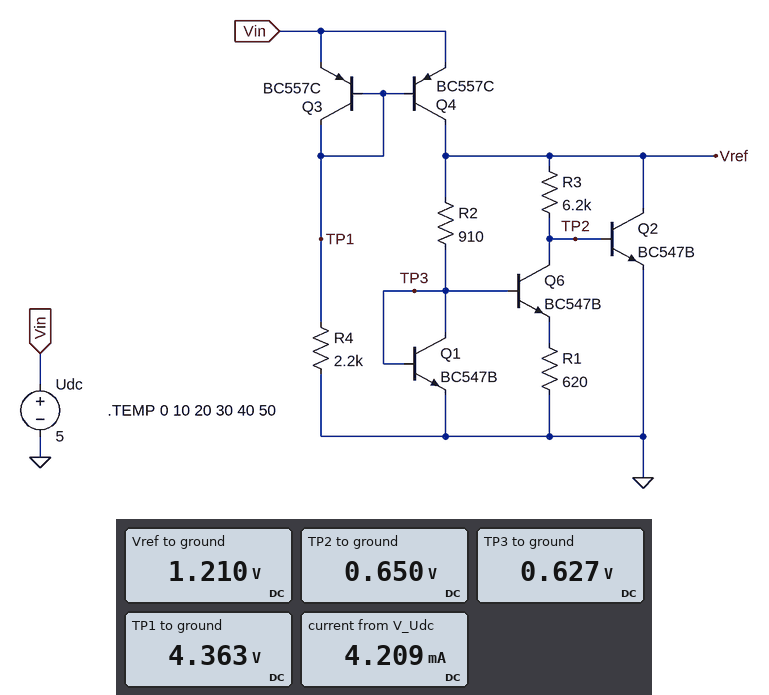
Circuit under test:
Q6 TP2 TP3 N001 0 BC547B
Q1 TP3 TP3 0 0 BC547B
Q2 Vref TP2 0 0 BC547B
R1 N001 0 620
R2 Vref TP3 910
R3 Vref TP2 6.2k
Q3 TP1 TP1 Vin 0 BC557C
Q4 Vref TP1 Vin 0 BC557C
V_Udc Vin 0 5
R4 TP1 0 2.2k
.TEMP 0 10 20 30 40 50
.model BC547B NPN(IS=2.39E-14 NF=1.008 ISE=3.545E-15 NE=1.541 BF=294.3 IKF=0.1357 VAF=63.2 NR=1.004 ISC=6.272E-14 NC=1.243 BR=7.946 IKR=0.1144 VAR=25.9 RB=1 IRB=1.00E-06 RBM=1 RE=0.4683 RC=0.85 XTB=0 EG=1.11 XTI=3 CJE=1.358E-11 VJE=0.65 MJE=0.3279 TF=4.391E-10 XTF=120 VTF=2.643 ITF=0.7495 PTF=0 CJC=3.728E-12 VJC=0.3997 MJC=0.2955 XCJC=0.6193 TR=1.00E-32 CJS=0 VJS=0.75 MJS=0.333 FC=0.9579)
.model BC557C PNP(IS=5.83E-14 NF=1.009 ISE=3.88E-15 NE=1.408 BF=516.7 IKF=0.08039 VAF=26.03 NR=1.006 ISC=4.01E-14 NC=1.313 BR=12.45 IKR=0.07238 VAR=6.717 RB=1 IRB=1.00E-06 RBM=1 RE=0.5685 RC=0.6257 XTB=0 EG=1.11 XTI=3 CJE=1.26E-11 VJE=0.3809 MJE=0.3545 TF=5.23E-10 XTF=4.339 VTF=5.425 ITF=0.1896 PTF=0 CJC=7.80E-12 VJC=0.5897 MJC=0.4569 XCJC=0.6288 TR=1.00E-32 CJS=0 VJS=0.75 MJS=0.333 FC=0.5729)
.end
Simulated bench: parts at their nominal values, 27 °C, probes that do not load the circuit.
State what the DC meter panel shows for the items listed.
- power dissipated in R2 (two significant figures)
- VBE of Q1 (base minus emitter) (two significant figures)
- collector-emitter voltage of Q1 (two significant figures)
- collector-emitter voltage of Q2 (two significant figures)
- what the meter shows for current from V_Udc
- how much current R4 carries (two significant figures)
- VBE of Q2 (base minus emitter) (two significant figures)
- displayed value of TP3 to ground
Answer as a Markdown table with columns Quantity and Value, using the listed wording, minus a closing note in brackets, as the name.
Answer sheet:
| Quantity | Value |
|---|---|
| power dissipated in R2 | 370 µW |
| VBE of Q1 (base minus emitter) | 630 mV |
| collector-emitter voltage of Q1 | 630 mV |
| collector-emitter voltage of Q2 | 1.2 V |
| what the meter shows for current from V_Udc | 4.209 mA |
| how much current R4 carries | 2.0 mA |
| VBE of Q2 (base minus emitter) | 650 mV |
| displayed value of TP3 to ground | 0.627 V |
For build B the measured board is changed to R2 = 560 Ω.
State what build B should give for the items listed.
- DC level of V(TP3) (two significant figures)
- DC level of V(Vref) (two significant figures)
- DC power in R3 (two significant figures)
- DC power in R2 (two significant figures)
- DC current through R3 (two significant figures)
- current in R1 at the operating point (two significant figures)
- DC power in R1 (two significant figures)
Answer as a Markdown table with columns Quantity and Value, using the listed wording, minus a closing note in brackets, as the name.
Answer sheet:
| Quantity | Value |
|---|---|
| DC level of V(TP3) | 640 mV |
| DC level of V(Vref) | 1.3 V |
| DC power in R3 | 70 µW |
| DC power in R2 | 760 µW |
| DC current through R3 | 110 µA |
| current in R1 at the operating point | 100 µA |
| DC power in R1 | 6.6 µW |
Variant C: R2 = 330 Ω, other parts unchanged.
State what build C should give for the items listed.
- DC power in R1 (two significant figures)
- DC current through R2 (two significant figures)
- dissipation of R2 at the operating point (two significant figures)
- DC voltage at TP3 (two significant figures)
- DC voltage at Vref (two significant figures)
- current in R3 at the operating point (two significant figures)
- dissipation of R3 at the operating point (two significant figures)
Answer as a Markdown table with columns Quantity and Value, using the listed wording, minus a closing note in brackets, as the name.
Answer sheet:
| Quantity | Value |
|---|---|
| DC power in R1 | 9.0 µW |
| DC current through R2 | 2.0 mA |
| dissipation of R2 at the operating point | 1.3 mW |
| DC voltage at TP3 | 660 mV |
| DC voltage at Vref | 1.3 V |
| current in R3 at the operating point | 120 µA |
| dissipation of R3 at the operating point | 90 µW |
